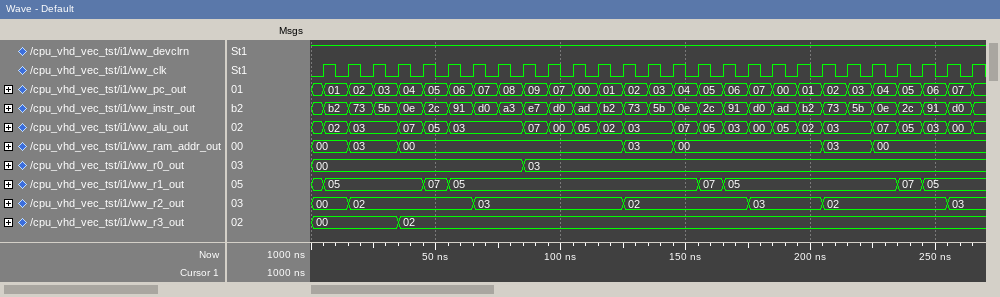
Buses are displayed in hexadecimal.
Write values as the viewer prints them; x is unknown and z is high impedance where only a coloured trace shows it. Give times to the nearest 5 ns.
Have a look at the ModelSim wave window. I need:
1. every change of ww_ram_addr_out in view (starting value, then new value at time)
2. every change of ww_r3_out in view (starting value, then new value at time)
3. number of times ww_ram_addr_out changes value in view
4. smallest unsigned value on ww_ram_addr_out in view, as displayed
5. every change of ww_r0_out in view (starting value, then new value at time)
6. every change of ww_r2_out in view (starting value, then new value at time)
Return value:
00, 03 at 15 ns, 00 at 35 ns, 03 at 125 ns, 00 at 145 ns, 03 at 205 ns, 00 at 225 ns
00, 02 at 35 ns
6
00
00, 03 at 85 ns
00, 02 at 15 ns, 03 at 65 ns, 02 at 125 ns, 03 at 175 ns, 02 at 205 ns, 03 at 255 ns
